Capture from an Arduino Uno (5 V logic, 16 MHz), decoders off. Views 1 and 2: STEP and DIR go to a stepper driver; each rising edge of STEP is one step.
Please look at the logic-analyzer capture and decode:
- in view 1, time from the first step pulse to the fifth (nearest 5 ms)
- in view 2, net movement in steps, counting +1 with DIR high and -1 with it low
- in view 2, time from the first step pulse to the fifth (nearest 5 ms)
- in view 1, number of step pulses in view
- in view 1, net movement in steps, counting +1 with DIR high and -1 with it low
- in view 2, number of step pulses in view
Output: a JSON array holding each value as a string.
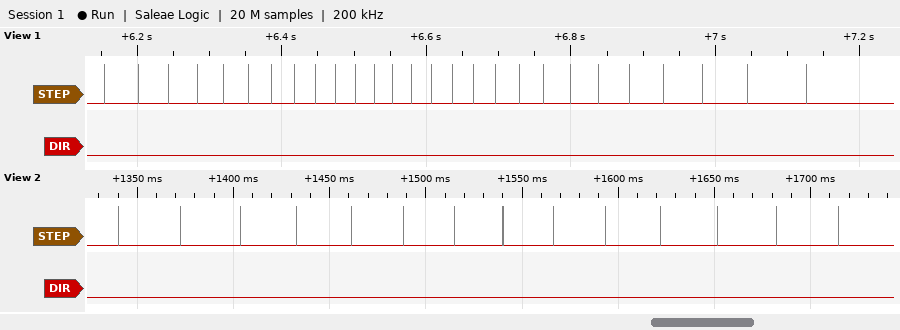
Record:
["165 ms", "-14", "120 ms", "27", "-27", "14"]
